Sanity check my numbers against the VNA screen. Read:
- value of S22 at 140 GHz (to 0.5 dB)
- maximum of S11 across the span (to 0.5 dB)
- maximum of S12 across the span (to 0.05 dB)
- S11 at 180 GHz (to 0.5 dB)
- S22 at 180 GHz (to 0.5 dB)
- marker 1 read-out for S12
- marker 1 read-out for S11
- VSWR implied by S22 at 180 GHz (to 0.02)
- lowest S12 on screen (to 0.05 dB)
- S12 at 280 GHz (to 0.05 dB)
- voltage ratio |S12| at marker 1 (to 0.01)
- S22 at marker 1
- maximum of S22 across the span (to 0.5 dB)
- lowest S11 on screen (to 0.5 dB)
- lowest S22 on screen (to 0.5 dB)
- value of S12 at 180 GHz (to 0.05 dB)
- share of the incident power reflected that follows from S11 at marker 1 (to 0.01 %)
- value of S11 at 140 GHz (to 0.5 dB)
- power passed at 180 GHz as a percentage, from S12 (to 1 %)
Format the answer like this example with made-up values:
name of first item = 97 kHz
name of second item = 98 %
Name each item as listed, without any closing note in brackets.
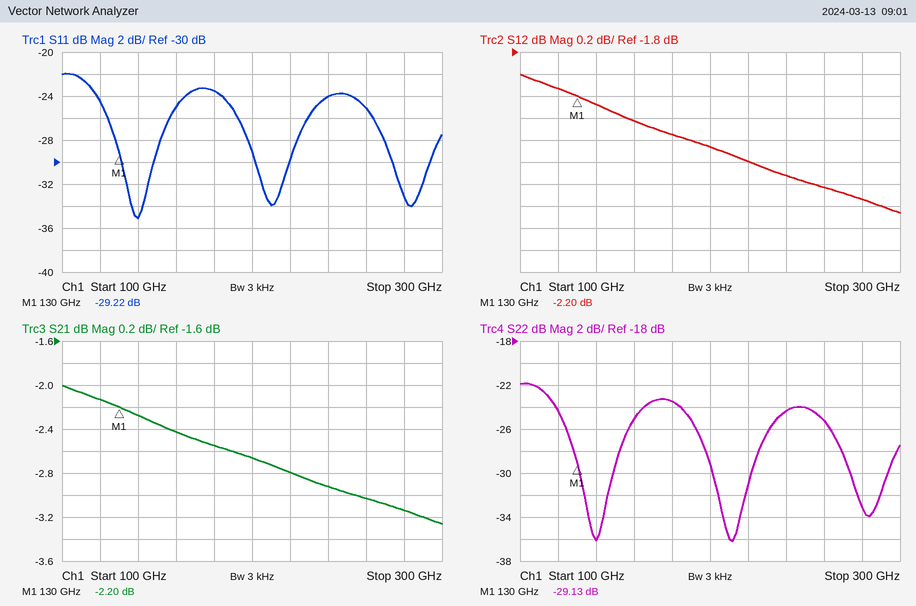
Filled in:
value of S22 at 140 GHz = -36.0 dB
maximum of S11 across the span = -22.0 dB
maximum of S12 across the span = -2.00 dB
S11 at 180 GHz = -23.5 dB
S22 at 180 GHz = -23.5 dB
marker 1 read-out for S12 = -2.20 dB
marker 1 read-out for S11 = -29.22 dB
VSWR implied by S22 at 180 GHz = 1.14
lowest S12 on screen = -3.25 dB
S12 at 280 GHz = -3.15 dB
voltage ratio |S12| at marker 1 = 0.78
S22 at marker 1 = -29.13 dB
maximum of S22 across the span = -22.0 dB
lowest S11 on screen = -35.0 dB
lowest S22 on screen = -36.0 dB
value of S12 at 180 GHz = -2.55 dB
share of the incident power reflected that follows from S11 at marker 1 = 0.12 %
value of S11 at 140 GHz = -35.0 dB
power passed at 180 GHz as a percentage, from S12 = 56 %
